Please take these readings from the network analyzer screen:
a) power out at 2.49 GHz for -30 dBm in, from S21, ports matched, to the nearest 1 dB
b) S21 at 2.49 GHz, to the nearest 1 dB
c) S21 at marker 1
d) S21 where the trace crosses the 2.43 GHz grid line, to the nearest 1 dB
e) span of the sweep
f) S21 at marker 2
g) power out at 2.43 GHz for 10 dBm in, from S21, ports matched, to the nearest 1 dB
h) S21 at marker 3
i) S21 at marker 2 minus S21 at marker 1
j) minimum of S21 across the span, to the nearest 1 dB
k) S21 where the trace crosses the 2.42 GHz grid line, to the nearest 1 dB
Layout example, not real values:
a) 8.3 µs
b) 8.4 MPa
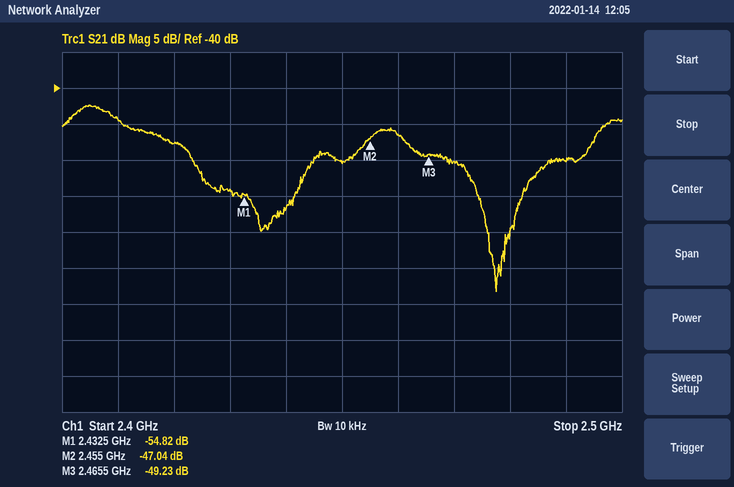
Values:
a) -80 dBm
b) -50 dB
c) -54.82 dB
d) -54 dB
e) 100 MHz
f) -47.04 dB
g) -44 dBm
h) -49.23 dB
i) 7.78 dB
j) -68 dB
k) -48 dB
